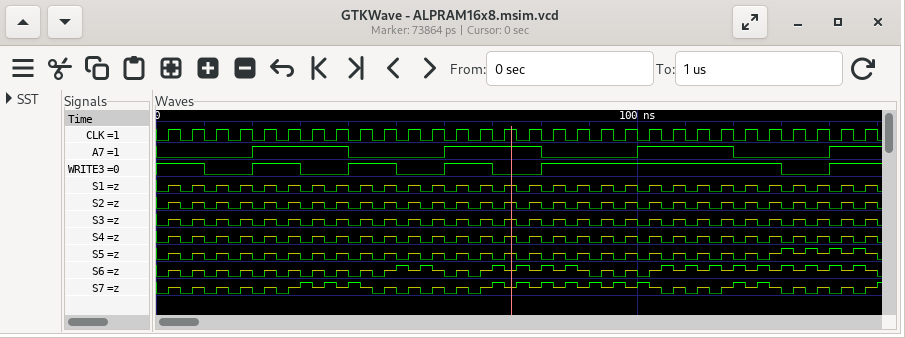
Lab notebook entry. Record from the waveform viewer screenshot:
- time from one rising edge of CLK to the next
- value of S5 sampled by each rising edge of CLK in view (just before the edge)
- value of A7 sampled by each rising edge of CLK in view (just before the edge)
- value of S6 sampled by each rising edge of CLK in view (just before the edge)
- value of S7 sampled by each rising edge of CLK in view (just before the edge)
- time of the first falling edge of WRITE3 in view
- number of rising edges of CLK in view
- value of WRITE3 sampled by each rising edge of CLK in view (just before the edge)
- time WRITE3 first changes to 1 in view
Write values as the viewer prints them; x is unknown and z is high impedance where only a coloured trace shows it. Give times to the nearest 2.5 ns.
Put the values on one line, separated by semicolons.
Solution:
5 ns; 0 0 0 0 0 0 0 0 0 0 0 0 0 0 0 0 0 0 0 0 0 0 0 0 0 0 1 1 1 1; 0 0 0 0 1 1 1 1 0 0 0 0 1 1 1 1 0 0 0 0 1 1 1 1 0 0 0 0 1 1; 0 0 0 0 0 0 0 0 0 0 1 1 0 0 1 1 1 1 0 0 0 1 1 1 1 1 1 1 1 1; 0 0 0 0 0 0 1 1 1 0 0 0 0 0 1 1 1 1 1 1 1 0 0 0 1 1 0 0 0 0; 10 ns; 30; 1 1 0 0 1 1 0 0 1 1 0 0 1 1 0 0 1 1 1 1 1 1 1 1 1 1 0 0 1 1; 20 ns
